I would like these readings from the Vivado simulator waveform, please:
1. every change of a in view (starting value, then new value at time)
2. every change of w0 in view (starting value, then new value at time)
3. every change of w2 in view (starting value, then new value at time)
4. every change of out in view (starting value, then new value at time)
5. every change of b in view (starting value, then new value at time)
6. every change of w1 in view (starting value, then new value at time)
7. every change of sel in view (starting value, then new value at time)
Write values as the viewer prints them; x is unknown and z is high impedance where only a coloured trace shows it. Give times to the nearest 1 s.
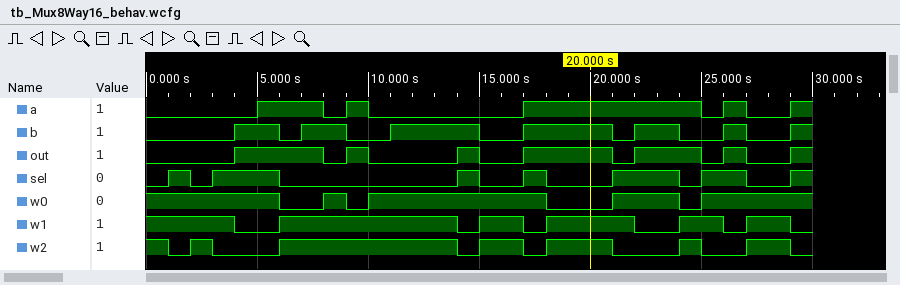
0, 1 at 5 s, 0 at 8 s, 1 at 9 s, 0 at 10 s, 1 at 17 s, 0 at 25 s, 1 at 26 s, 0 at 27 s, 1 at 29 s
1, 0 at 6 s, 1 at 8 s, 0 at 9 s, 1 at 10 s, 0 at 18 s, 1 at 21 s, 0 at 24 s, 1 at 25 s
1, 0 at 1 s, 1 at 2 s, 0 at 3 s, 1 at 6 s, 0 at 14 s, 1 at 15 s, 0 at 17 s, 1 at 18 s, 0 at 21 s, 1 at 24 s, 0 at 25 s, 1 at 27 s, 0 at 29 s
0, 1 at 4 s, 0 at 8 s, 1 at 9 s, 0 at 10 s, 1 at 14 s, 0 at 15 s, 1 at 17 s, 0 at 21 s, 1 at 22 s, 0 at 25 s, 1 at 26 s, 0 at 27 s, 1 at 29 s
0, 1 at 4 s, 0 at 6 s, 1 at 7 s, 0 at 9 s, 1 at 11 s, 0 at 15 s, 1 at 17 s, 0 at 21 s, 1 at 22 s, 0 at 24 s, 1 at 26 s, 0 at 27 s, 1 at 29 s
1, 0 at 4 s, 1 at 6 s, 0 at 14 s, 1 at 15 s, 0 at 17 s, 1 at 18 s, 0 at 22 s, 1 at 24 s, 0 at 26 s, 1 at 27 s, 0 at 29 s
0, 1 at 1 s, 0 at 2 s, 1 at 3 s, 0 at 6 s, 1 at 14 s, 0 at 15 s, 1 at 17 s, 0 at 18 s, 1 at 21 s, 0 at 24 s, 1 at 25 s, 0 at 27 s, 1 at 29 s
